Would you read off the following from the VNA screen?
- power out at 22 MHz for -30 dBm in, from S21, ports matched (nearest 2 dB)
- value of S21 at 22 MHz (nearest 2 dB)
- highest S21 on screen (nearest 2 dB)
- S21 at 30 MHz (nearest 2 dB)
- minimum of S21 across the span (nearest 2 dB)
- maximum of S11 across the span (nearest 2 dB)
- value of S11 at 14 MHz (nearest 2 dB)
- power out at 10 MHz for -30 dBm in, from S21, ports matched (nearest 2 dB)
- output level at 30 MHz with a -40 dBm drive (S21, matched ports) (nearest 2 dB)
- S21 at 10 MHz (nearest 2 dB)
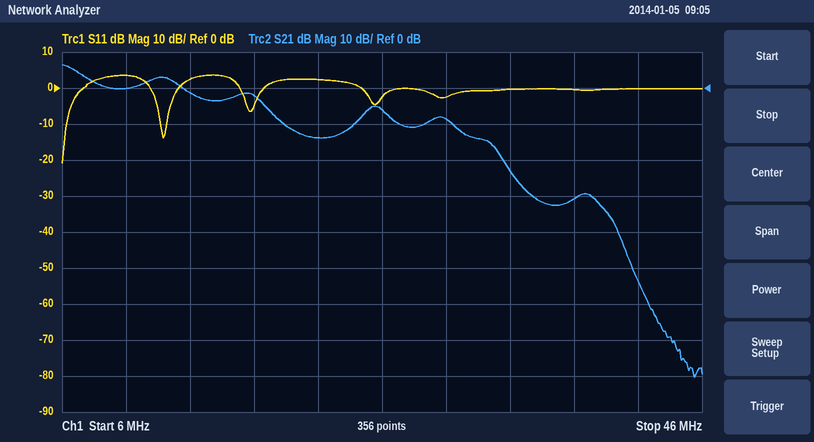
-44 dBm
-14 dB
6 dB
-8 dB
-80 dB
4 dB
2 dB
-30 dBm
-48 dBm
0 dB
